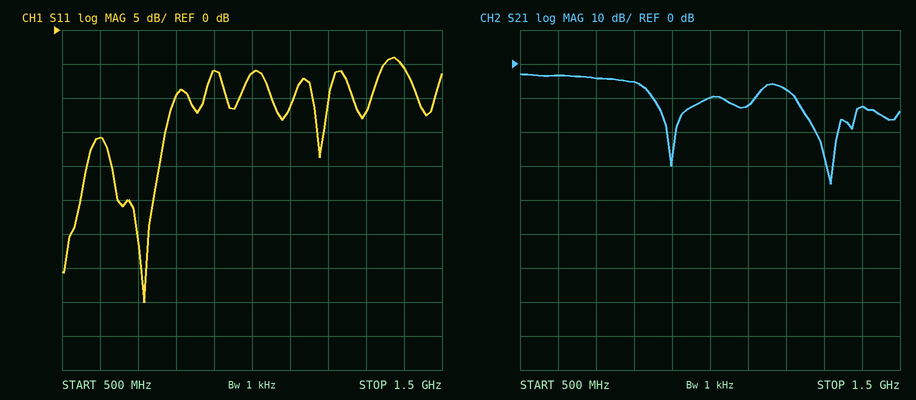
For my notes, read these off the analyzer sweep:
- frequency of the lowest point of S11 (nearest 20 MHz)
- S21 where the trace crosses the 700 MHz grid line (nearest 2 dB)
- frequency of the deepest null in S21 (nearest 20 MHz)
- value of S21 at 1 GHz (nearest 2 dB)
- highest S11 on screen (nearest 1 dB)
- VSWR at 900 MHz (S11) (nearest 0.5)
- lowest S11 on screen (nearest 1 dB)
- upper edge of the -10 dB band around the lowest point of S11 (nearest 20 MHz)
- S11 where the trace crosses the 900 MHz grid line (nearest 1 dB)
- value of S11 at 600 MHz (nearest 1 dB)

720 MHz
-4 dB
1.32 GHz
-10 dB
-4 dB
3.0
-40 dB
800 MHz
-6 dB
-16 dB
